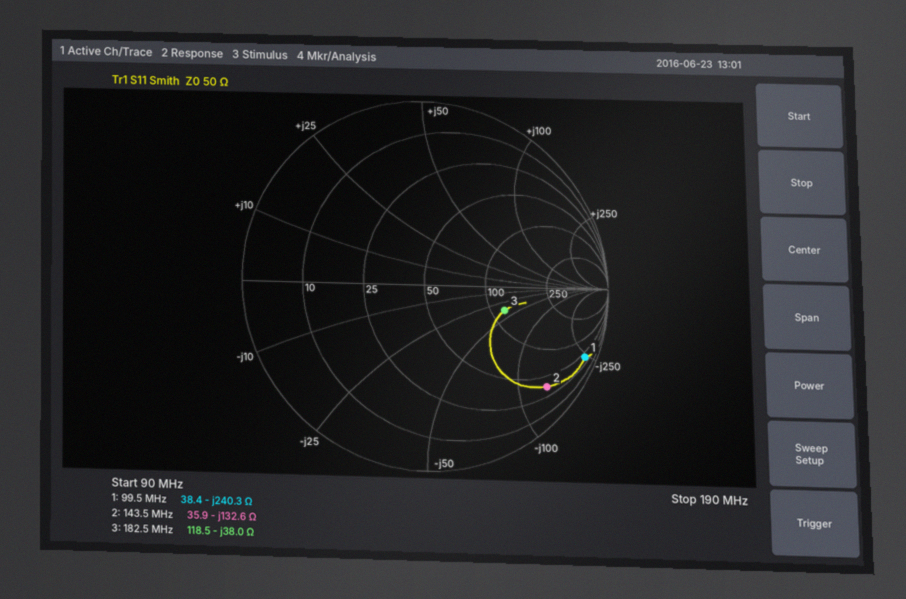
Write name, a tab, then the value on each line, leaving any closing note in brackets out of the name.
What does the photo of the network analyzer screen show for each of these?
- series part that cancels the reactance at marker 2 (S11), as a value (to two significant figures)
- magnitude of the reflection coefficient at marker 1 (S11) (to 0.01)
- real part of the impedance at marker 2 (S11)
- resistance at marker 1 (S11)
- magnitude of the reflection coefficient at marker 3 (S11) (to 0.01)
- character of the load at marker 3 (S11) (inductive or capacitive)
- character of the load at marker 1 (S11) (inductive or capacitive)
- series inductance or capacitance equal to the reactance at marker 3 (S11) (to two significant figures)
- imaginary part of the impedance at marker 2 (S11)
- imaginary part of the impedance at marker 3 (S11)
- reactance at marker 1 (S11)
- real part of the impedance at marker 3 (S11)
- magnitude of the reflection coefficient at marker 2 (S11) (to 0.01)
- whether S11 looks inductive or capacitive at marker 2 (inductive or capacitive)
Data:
series part that cancels the reactance at marker 2 (S11), as a value	150 nH
magnitude of the reflection coefficient at marker 1 (S11)	0.94
real part of the impedance at marker 2	35.9 Ω
resistance at marker 1	38.4 Ω
magnitude of the reflection coefficient at marker 3 (S11)	0.45
character of the load at marker 3 (S11)	capacitive
character of the load at marker 1 (S11)	capacitive
series inductance or capacitance equal to the reactance at marker 3 (S11)	23 pF
imaginary part of the impedance at marker 2	-132.6 Ω
imaginary part of the impedance at marker 3	-38.0 Ω
reactance at marker 1	-240.3 Ω
real part of the impedance at marker 3	118.5 Ω
magnitude of the reflection coefficient at marker 2 (S11)	0.84
whether S11 looks inductive or capacitive at marker 2	capacitive
